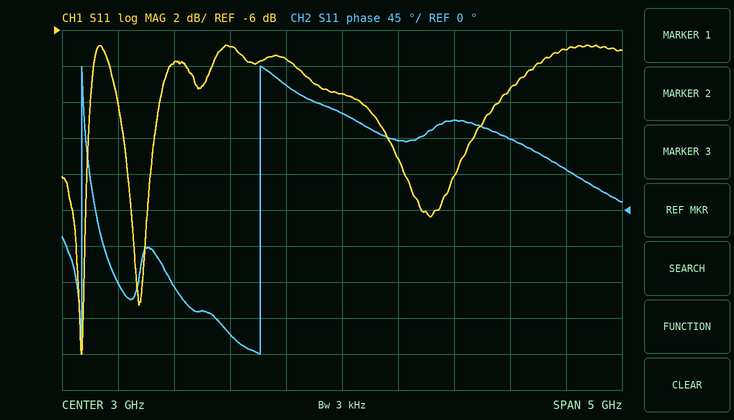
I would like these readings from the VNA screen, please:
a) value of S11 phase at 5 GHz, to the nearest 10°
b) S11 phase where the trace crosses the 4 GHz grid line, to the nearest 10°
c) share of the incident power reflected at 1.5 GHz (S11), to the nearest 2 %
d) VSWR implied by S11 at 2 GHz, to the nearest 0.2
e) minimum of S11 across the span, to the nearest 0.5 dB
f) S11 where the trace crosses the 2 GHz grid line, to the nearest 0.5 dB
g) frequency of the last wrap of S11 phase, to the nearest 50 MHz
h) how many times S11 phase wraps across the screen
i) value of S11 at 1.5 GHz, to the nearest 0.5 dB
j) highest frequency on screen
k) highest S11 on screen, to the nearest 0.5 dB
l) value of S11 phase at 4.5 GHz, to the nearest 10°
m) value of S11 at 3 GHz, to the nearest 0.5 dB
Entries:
50°
110°
16 %
2.6
-24.0 dB
-7.0 dB
2.25 GHz
2
-8.0 dB
5.5 GHz
-7.0 dB
90°
-9.5 dB
